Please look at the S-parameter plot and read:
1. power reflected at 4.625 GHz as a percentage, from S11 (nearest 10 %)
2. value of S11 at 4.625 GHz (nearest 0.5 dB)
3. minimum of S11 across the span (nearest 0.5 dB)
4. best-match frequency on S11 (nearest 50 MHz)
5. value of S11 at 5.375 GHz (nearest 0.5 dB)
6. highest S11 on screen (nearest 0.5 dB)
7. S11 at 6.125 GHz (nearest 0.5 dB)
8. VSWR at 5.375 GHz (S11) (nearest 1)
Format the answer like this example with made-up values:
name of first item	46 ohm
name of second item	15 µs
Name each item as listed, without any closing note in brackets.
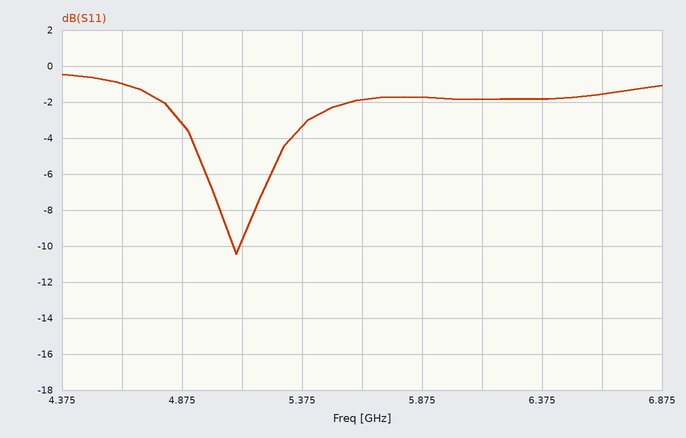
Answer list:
power reflected at 4.625 GHz as a percentage, from S11	80 %
value of S11 at 4.625 GHz	-1.0 dB
minimum of S11 across the span	-10.5 dB
best-match frequency on S11	5.10 GHz
value of S11 at 5.375 GHz	-3.5 dB
highest S11 on screen	-0.5 dB
S11 at 6.125 GHz	-2.0 dB
VSWR at 5.375 GHz (S11)	5
